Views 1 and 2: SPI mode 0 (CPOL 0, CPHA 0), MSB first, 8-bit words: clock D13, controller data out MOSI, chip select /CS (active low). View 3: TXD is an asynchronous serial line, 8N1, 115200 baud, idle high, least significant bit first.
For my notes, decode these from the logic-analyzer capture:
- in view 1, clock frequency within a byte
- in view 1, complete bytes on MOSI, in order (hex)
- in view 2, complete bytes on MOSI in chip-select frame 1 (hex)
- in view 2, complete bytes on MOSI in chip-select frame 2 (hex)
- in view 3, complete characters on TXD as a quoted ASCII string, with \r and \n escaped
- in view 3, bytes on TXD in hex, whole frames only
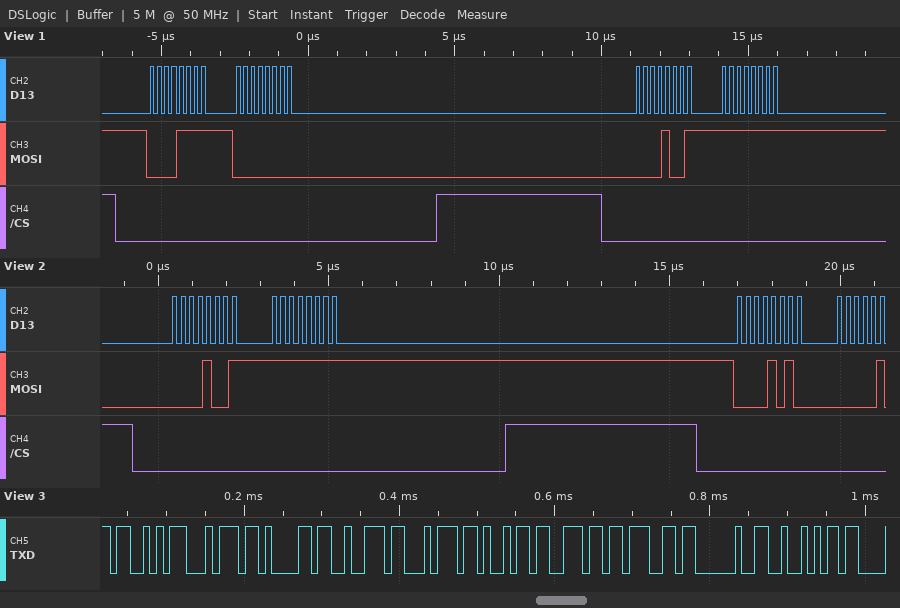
4 MHz
0x0F 0x00 0x09 0xFF
09 FF
0A
"Starting R"
53 74 61 72 74 69 6E 67 20 52
